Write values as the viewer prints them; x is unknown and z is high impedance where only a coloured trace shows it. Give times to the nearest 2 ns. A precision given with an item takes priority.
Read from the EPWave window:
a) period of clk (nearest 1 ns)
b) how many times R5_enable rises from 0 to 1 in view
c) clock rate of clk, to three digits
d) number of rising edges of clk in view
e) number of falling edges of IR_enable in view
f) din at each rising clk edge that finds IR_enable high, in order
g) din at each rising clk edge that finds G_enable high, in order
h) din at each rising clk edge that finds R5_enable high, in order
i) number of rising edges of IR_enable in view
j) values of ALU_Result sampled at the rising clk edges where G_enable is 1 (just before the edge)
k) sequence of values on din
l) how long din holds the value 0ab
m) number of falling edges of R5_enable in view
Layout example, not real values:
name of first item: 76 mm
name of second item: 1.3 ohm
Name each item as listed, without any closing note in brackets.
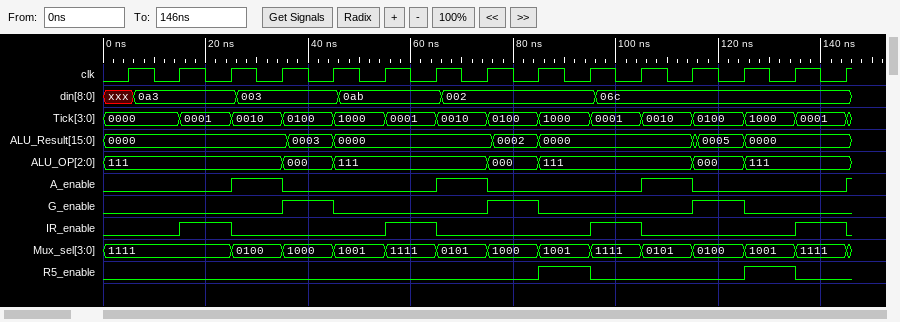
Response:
period of clk: 10 ns
how many times R5_enable rises from 0 to 1 in view: 2
clock rate of clk, to three digits: 100 MHz
number of rising edges of clk in view: 15
number of falling edges of IR_enable in view: 4
din at each rising clk edge that finds IR_enable high, in order: 0a3, 0ab, 06c, 06c
din at each rising clk edge that finds G_enable high, in order: 003, 002, 06c
din at each rising clk edge that finds R5_enable high, in order: 002, 06c
number of rising edges of IR_enable in view: 4
values of ALU_Result sampled at the rising clk edges where G_enable is 1: 0003, 0002, 0005
sequence of values on din: xxx, 0a3, 003, 0ab, 002, 06c
how long din holds the value 0ab: 20 ns
number of falling edges of R5_enable in view: 2
